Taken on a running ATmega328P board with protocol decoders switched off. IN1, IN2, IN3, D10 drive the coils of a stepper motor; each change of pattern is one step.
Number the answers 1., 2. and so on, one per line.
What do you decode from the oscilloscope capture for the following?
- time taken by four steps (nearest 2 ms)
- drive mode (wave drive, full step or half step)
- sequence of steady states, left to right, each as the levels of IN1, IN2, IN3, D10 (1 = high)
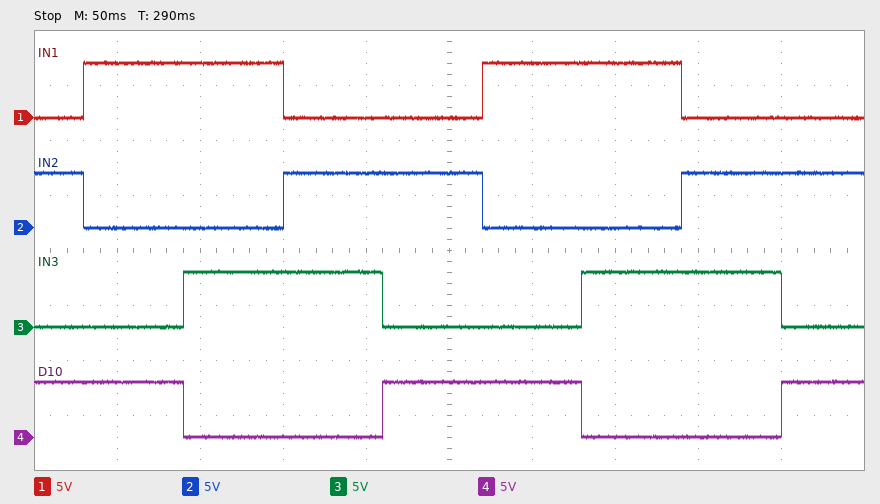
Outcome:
1. 240 ms
2. full step
3. 0101 1001 1010 0110 0101 1001 1010 0110 0101
